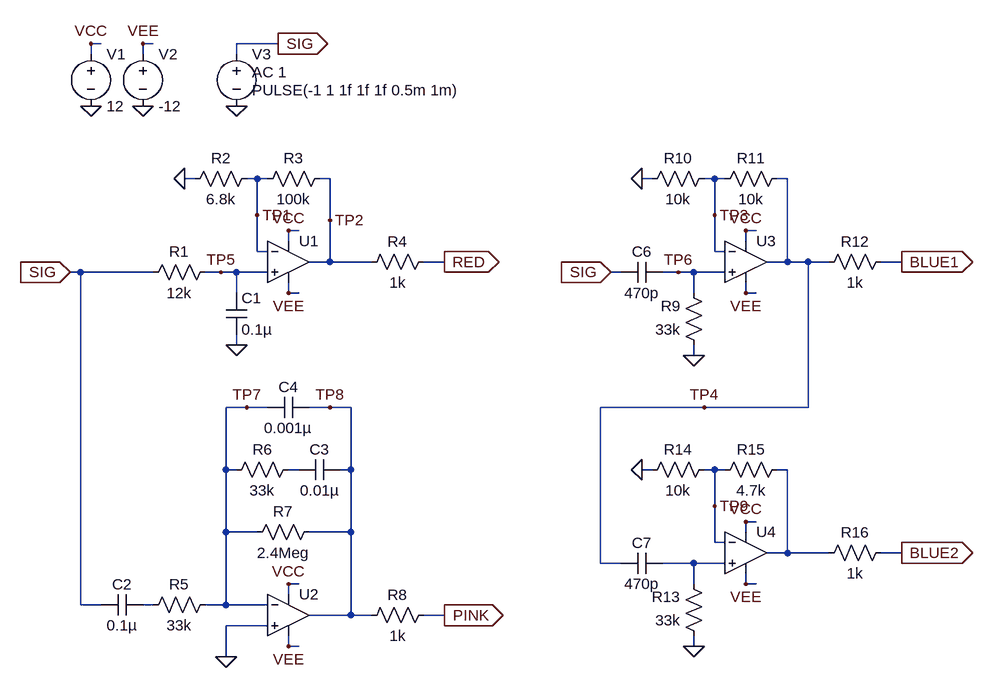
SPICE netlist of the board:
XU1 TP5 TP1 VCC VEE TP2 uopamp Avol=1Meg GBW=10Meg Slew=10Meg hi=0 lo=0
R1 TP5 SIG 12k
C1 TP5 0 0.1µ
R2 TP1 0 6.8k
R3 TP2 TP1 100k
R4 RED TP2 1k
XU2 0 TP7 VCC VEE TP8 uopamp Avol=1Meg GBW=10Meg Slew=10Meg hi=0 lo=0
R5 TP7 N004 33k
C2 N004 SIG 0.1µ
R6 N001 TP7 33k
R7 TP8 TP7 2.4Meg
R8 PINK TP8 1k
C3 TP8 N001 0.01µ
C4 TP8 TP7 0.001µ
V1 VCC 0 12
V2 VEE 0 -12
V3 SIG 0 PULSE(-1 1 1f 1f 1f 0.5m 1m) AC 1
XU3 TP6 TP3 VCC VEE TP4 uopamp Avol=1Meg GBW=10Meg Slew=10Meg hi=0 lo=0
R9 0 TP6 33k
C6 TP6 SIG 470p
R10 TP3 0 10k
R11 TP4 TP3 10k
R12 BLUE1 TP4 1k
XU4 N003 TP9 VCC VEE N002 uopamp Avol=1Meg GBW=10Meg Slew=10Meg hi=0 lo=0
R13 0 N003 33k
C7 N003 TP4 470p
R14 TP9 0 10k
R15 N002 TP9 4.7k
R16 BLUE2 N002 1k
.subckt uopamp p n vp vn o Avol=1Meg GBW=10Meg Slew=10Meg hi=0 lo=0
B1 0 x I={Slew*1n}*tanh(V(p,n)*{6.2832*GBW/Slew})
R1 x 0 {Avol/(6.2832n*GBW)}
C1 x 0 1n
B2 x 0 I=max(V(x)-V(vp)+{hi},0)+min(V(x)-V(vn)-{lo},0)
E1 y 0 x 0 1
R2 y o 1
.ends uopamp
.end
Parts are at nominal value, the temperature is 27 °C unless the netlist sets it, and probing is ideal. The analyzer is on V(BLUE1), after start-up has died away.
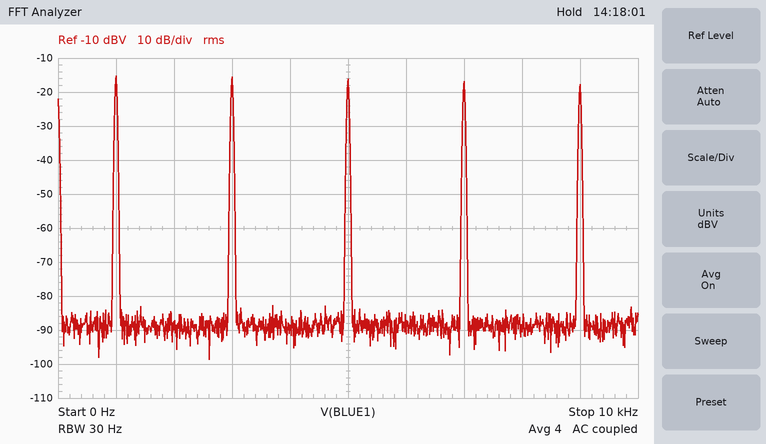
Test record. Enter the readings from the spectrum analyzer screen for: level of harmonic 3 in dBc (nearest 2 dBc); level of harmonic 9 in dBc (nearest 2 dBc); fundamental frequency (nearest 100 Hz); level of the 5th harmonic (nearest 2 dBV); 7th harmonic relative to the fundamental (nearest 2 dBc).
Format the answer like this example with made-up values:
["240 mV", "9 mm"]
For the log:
["0 dBc", "-2 dBc", "1.0 kHz", "-16 dBV", "-2 dBc"]
